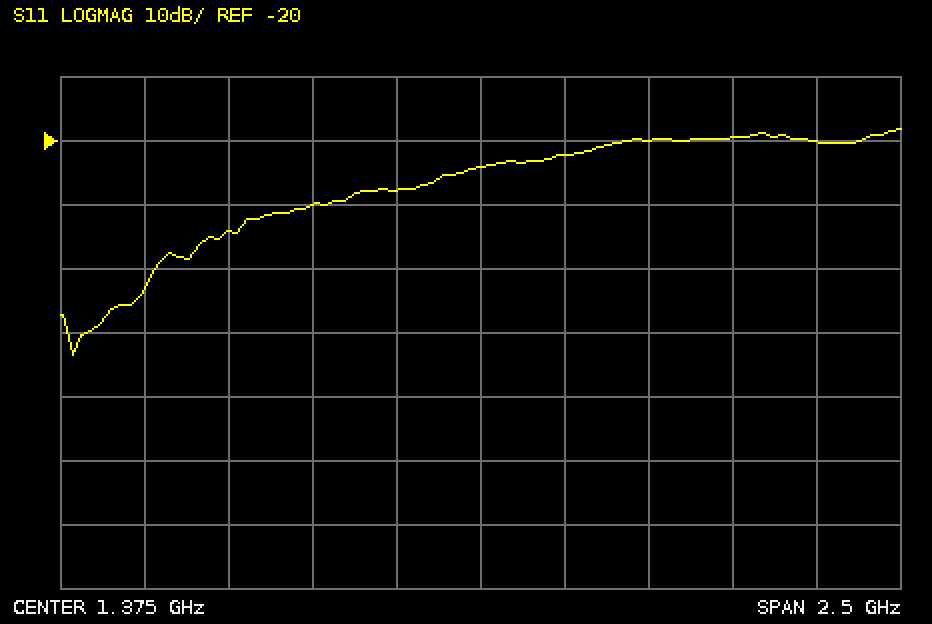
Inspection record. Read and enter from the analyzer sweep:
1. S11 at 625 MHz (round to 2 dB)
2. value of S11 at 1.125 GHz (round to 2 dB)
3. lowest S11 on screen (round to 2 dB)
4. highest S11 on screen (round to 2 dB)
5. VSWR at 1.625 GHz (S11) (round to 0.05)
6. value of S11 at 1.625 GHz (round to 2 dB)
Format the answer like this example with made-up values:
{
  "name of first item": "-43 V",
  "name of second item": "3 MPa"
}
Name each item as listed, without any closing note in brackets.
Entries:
{
  "S11 at 625 MHz": "-34 dB",
  "value of S11 at 1.125 GHz": "-28 dB",
  "lowest S11 on screen": "-54 dB",
  "highest S11 on screen": "-18 dB",
  "VSWR at 1.625 GHz (S11)": "1.15",
  "value of S11 at 1.625 GHz": "-22 dB"
}
